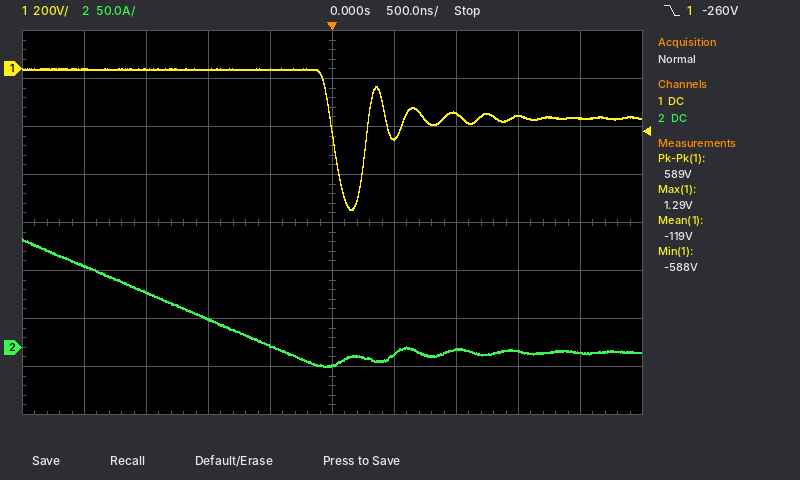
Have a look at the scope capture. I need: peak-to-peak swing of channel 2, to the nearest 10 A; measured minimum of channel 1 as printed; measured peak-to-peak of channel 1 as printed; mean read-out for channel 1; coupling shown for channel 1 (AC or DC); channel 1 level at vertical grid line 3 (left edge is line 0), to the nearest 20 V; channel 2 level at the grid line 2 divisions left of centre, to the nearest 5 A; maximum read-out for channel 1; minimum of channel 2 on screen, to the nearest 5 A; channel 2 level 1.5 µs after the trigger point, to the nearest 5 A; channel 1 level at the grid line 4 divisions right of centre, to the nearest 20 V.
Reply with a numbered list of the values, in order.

1. 130 A
2. -588 V
3. 589 V
4. -119 V
5. DC
6. 0 V
7. 30 A
8. 1.29 V
9. -20 A
10. -5 A
11. -200 V
